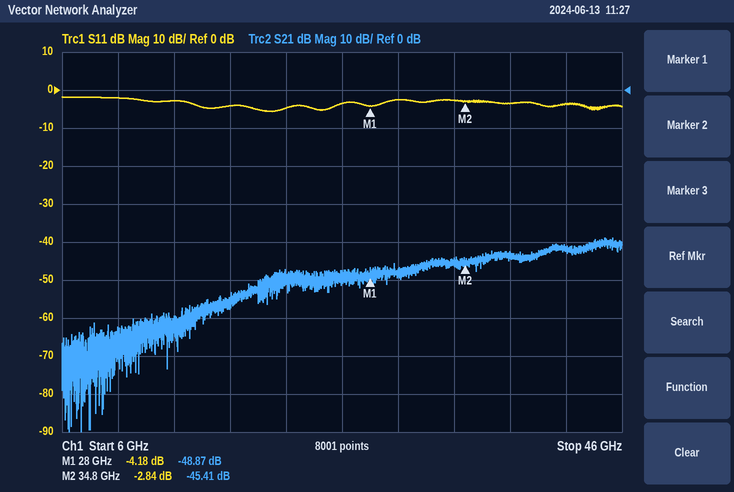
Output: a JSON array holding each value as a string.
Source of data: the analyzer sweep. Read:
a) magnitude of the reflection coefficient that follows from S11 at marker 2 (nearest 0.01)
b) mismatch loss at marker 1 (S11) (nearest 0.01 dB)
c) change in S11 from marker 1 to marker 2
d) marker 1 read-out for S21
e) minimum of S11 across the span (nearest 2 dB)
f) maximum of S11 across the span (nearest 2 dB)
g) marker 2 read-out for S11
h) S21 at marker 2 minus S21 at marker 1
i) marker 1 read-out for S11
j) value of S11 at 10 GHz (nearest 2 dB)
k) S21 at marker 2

["0.72", "2.09 dB", "1.34 dB", "-48.87 dB", "-6 dB", "-2 dB", "-2.84 dB", "3.46 dB", "-4.18 dB", "-2 dB", "-45.41 dB"]
